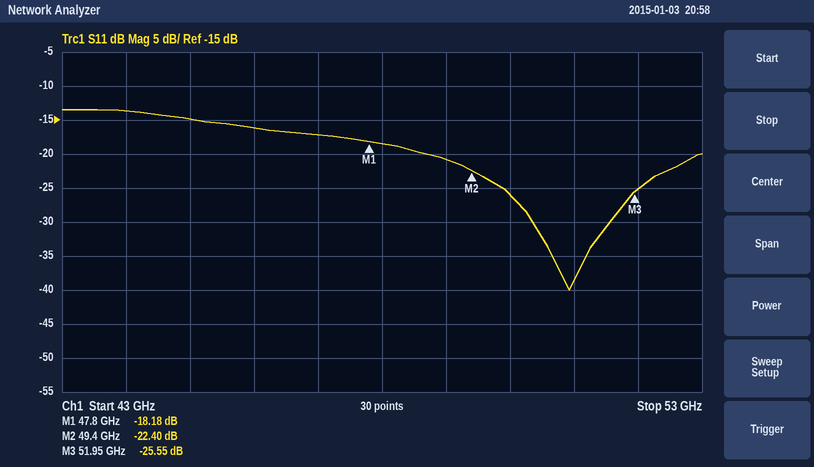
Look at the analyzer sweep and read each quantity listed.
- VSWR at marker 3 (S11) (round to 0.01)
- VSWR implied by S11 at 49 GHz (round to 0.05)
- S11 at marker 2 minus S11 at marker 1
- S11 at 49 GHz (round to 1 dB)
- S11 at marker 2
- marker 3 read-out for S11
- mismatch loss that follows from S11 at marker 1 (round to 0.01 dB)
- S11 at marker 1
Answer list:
1.11
1.20
-4.22 dB
-21 dB
-22.40 dB
-25.55 dB
0.07 dB
-18.18 dB
